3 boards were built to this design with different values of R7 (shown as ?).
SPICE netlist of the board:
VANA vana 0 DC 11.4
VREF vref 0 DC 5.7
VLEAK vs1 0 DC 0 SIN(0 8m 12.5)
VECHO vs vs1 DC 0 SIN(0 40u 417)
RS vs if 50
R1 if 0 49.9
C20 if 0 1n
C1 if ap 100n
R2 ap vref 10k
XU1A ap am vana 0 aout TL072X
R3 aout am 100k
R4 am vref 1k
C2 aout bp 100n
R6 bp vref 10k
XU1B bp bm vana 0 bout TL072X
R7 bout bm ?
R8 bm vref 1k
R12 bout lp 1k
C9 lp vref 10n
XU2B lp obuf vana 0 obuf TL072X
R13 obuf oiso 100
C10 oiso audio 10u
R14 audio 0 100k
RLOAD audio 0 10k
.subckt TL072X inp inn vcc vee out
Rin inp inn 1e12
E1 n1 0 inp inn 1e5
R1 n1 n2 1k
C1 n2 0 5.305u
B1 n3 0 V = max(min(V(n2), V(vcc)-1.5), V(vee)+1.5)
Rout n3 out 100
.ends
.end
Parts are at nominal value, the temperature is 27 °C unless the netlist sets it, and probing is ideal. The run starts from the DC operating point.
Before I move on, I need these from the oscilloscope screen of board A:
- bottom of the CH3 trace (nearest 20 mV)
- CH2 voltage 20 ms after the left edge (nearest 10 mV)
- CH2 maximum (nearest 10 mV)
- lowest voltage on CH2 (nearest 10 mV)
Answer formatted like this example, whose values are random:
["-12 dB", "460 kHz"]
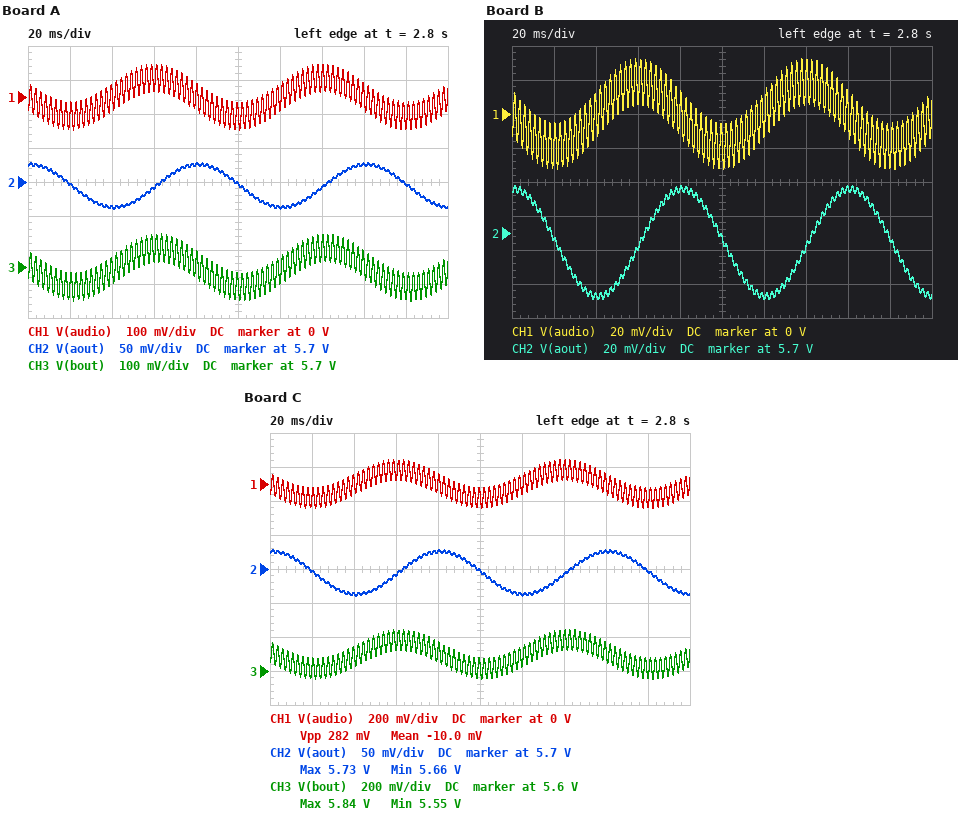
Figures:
["5.60 V", "5.70 V", "5.73 V", "5.66 V"]
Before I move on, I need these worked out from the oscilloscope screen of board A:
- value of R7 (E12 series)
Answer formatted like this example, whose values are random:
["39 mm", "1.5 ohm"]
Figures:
["22 kΩ"]
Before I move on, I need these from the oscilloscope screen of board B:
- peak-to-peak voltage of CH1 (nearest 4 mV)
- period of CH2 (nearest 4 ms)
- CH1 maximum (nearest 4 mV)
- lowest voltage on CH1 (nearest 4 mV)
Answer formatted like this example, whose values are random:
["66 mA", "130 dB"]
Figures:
["64 mV", "80 ms", "32 mV", "-32 mV"]
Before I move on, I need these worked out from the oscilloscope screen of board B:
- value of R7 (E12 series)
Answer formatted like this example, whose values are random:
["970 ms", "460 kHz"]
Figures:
["6.8 kΩ"]
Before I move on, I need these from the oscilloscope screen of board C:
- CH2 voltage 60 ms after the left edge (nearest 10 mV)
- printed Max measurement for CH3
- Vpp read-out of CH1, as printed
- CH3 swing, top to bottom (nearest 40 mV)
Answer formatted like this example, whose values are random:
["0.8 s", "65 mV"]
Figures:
["5.69 V", "5.84 V", "282 mV", "280 mV"]
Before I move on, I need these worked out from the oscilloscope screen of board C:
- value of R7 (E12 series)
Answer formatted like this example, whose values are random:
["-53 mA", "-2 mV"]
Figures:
["33 kΩ"]
